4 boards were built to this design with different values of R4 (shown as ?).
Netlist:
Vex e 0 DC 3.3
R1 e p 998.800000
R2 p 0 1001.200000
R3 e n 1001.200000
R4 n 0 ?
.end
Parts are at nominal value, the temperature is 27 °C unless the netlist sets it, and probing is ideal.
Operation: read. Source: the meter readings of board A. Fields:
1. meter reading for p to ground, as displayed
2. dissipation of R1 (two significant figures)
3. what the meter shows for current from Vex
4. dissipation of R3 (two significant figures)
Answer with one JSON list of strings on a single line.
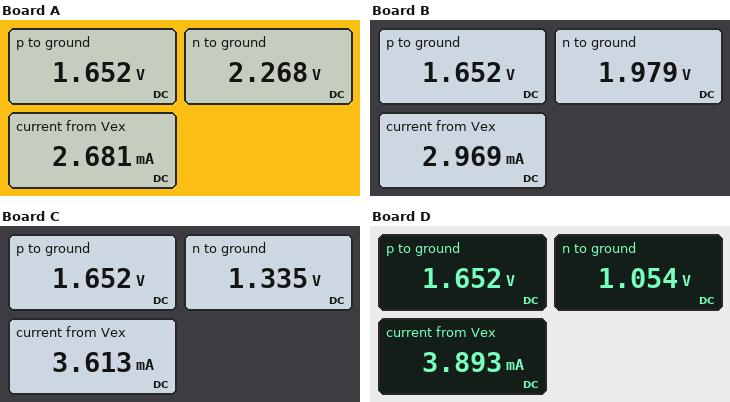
["1.652 V", "2.7 mW", "2.681 mA", "1.1 mW"]
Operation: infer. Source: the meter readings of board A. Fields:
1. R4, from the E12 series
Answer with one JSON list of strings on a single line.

["2.2 kΩ"]
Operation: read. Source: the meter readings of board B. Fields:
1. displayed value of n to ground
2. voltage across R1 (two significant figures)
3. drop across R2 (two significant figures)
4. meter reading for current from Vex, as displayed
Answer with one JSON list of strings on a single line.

["1.979 V", "1.6 V", "1.7 V", "2.969 mA"]
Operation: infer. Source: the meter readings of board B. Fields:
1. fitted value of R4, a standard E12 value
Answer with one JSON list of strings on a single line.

["1.5 kΩ"]
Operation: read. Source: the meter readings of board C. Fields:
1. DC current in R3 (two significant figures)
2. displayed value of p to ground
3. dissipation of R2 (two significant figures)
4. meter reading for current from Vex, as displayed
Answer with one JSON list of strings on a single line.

["2.0 mA", "1.652 V", "2.7 mW", "3.613 mA"]
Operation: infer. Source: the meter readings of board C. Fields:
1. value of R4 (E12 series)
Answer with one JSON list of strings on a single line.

["680 Ω"]
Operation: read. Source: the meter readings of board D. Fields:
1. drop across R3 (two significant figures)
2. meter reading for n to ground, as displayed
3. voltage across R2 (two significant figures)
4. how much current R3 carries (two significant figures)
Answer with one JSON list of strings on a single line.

["2.2 V", "1.054 V", "1.7 V", "2.2 mA"]
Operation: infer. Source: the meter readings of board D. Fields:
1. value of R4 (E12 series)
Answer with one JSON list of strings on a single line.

["470 Ω"]
